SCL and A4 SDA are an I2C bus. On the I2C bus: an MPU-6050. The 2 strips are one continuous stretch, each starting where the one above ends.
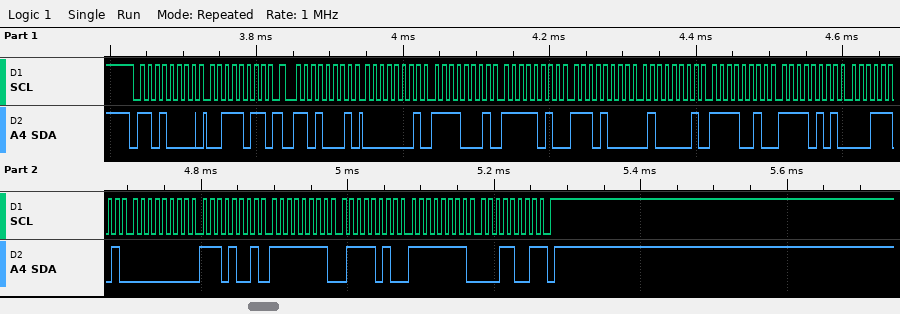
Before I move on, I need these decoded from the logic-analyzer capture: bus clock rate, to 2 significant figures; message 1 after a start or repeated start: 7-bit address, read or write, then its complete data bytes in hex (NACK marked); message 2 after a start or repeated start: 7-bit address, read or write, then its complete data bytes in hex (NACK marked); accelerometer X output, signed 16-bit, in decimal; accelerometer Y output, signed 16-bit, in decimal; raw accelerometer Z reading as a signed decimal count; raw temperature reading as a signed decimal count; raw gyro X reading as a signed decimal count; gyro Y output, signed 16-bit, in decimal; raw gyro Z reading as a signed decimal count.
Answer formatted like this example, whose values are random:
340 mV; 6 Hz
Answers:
100 kHz; 0x68 write: 3B; 0x68 read: 01 F1 FA E8 41 F2 F5 1D 00 E9 FF 7A FF 19 NACK; 497; -1304; 16882; -2787; 233; -134; -231
